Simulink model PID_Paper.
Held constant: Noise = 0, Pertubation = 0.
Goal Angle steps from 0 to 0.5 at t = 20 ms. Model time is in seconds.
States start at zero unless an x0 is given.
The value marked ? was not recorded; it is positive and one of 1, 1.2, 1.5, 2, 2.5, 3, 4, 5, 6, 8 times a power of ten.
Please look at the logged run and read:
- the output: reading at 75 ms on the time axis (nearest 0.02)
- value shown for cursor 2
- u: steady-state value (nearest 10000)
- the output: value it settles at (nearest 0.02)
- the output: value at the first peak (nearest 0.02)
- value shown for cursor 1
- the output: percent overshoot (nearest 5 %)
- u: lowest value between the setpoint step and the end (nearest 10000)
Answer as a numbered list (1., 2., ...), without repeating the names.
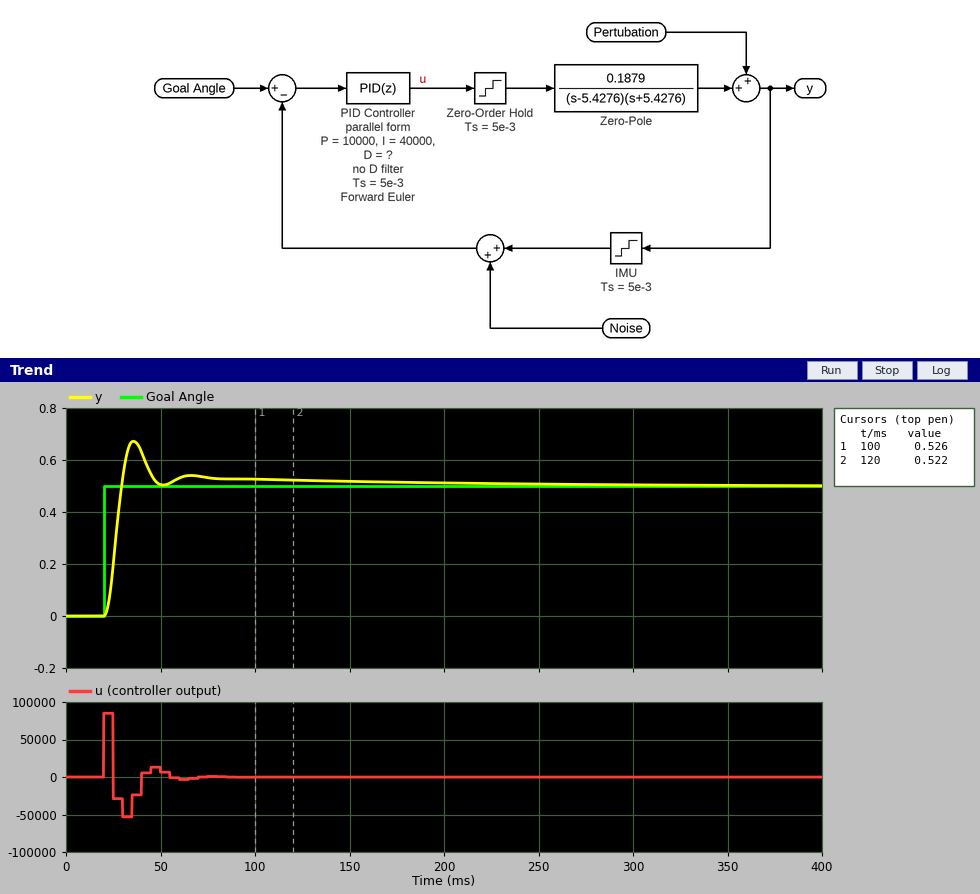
1. 0.54
2. 0.522
3. 0
4. 0.50
5. 0.68
6. 0.526
7. 35 %
8. -50000
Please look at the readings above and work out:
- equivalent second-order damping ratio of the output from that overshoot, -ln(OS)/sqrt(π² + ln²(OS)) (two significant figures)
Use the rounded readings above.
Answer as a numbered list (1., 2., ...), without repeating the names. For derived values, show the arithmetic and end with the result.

1. ln(0.35) = -1.050; 1.050 / sqrt(9.870 + 1.102) = 0.32
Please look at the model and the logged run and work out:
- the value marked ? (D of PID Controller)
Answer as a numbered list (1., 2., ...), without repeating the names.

1. 800
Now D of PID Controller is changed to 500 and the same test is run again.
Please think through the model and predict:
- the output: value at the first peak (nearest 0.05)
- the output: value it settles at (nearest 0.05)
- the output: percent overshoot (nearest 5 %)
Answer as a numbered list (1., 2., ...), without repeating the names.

1. 0.60
2. 0.50
3. 25 %
